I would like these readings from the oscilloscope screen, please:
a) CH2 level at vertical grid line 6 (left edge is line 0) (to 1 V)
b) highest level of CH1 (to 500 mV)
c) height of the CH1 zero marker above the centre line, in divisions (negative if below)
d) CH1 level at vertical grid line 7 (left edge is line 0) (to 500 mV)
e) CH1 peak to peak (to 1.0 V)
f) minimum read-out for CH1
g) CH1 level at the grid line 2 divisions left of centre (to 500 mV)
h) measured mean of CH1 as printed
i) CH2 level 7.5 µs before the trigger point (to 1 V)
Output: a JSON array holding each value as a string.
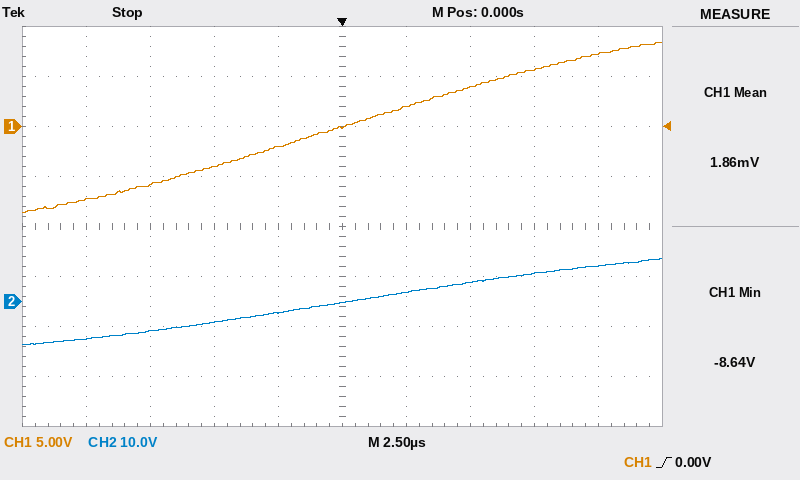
["2 V", "8.5 V", "+2.0 div", "4.0 V", "17.0 V", "-8.64 V", "-4.0 V", "1.86 mV", "-6 V"]
